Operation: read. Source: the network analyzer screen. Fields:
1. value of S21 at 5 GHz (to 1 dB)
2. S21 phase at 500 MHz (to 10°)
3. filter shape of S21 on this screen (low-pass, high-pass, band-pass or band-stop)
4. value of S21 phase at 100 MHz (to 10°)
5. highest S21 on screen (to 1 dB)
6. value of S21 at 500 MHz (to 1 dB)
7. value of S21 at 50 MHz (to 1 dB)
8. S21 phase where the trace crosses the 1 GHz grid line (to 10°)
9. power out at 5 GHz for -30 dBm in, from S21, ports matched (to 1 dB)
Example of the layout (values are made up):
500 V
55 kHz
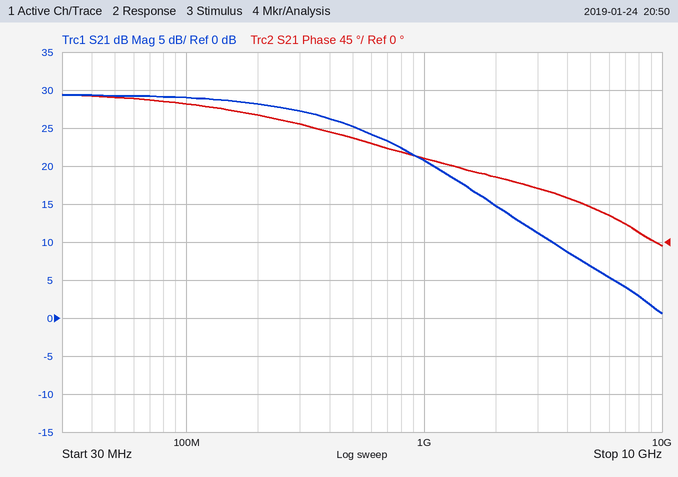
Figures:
7 dB
120°
low-pass
160°
29 dB
25 dB
29 dB
100°
-23 dBm
